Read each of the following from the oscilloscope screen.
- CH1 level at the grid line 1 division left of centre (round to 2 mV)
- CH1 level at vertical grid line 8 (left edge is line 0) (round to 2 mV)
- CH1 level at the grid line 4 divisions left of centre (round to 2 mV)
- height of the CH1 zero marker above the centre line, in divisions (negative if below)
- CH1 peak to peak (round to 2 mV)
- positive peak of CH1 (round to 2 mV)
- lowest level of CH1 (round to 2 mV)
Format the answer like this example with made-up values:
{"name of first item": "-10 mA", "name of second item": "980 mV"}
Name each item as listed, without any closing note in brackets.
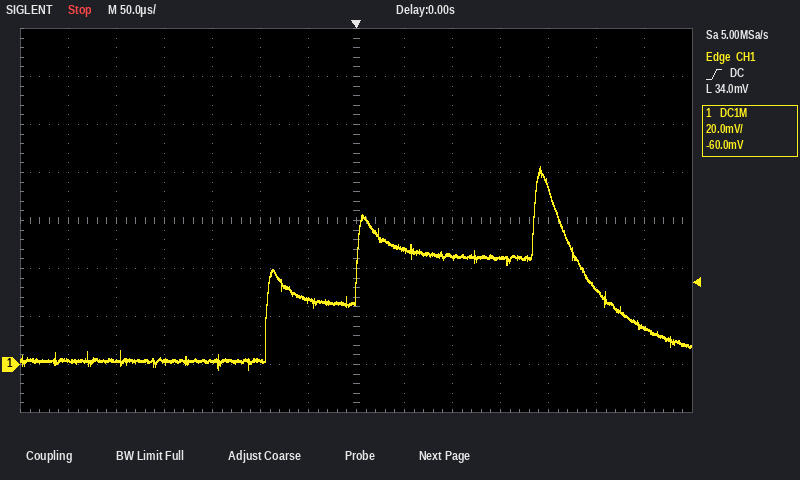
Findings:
{"CH1 level at the grid line 1 division left of centre": "26 mV", "CH1 level at vertical grid line 8 (left edge is line 0)": "48 mV", "CH1 level at the grid line 4 divisions left of centre": "2 mV", "height of the CH1 zero marker above the centre line, in divisions": "-3.0 div", "CH1 peak to peak": "84 mV", "positive peak of CH1": "82 mV", "lowest level of CH1": "-2 mV"}
